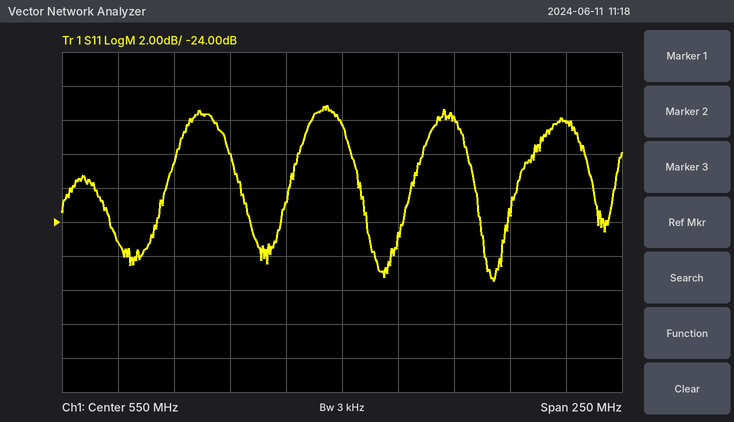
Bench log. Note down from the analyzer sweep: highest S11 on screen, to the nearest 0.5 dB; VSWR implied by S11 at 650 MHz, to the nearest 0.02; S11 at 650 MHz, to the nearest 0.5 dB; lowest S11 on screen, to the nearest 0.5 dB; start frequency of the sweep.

-17.0 dB
1.28
-18.0 dB
-27.5 dB
425 MHz
